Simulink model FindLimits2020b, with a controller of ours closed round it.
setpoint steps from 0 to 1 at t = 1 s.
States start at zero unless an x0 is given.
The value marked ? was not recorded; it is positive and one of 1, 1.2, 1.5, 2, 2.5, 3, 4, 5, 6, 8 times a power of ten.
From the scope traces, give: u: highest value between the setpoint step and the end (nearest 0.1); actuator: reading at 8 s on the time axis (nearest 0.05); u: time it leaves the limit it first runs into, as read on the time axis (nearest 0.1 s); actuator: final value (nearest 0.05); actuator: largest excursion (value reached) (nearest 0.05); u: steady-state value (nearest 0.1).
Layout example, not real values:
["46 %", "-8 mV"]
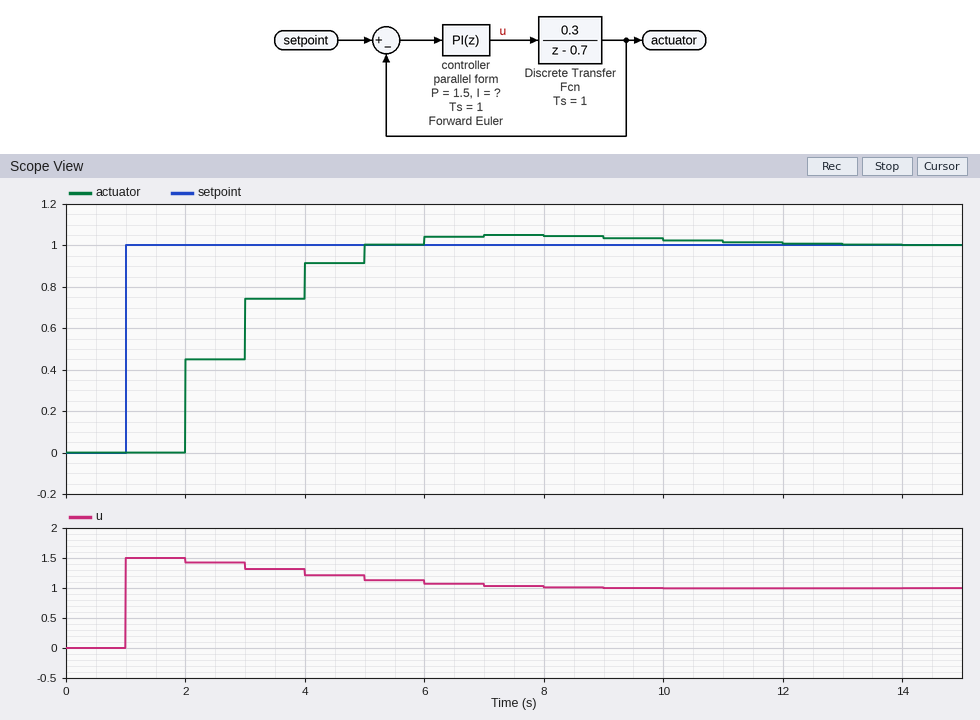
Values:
["1.5", "1.05", "2.0 s", "1.00", "1.05", "1.0"]
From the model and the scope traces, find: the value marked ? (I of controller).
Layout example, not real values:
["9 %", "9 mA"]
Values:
["0.6"]
